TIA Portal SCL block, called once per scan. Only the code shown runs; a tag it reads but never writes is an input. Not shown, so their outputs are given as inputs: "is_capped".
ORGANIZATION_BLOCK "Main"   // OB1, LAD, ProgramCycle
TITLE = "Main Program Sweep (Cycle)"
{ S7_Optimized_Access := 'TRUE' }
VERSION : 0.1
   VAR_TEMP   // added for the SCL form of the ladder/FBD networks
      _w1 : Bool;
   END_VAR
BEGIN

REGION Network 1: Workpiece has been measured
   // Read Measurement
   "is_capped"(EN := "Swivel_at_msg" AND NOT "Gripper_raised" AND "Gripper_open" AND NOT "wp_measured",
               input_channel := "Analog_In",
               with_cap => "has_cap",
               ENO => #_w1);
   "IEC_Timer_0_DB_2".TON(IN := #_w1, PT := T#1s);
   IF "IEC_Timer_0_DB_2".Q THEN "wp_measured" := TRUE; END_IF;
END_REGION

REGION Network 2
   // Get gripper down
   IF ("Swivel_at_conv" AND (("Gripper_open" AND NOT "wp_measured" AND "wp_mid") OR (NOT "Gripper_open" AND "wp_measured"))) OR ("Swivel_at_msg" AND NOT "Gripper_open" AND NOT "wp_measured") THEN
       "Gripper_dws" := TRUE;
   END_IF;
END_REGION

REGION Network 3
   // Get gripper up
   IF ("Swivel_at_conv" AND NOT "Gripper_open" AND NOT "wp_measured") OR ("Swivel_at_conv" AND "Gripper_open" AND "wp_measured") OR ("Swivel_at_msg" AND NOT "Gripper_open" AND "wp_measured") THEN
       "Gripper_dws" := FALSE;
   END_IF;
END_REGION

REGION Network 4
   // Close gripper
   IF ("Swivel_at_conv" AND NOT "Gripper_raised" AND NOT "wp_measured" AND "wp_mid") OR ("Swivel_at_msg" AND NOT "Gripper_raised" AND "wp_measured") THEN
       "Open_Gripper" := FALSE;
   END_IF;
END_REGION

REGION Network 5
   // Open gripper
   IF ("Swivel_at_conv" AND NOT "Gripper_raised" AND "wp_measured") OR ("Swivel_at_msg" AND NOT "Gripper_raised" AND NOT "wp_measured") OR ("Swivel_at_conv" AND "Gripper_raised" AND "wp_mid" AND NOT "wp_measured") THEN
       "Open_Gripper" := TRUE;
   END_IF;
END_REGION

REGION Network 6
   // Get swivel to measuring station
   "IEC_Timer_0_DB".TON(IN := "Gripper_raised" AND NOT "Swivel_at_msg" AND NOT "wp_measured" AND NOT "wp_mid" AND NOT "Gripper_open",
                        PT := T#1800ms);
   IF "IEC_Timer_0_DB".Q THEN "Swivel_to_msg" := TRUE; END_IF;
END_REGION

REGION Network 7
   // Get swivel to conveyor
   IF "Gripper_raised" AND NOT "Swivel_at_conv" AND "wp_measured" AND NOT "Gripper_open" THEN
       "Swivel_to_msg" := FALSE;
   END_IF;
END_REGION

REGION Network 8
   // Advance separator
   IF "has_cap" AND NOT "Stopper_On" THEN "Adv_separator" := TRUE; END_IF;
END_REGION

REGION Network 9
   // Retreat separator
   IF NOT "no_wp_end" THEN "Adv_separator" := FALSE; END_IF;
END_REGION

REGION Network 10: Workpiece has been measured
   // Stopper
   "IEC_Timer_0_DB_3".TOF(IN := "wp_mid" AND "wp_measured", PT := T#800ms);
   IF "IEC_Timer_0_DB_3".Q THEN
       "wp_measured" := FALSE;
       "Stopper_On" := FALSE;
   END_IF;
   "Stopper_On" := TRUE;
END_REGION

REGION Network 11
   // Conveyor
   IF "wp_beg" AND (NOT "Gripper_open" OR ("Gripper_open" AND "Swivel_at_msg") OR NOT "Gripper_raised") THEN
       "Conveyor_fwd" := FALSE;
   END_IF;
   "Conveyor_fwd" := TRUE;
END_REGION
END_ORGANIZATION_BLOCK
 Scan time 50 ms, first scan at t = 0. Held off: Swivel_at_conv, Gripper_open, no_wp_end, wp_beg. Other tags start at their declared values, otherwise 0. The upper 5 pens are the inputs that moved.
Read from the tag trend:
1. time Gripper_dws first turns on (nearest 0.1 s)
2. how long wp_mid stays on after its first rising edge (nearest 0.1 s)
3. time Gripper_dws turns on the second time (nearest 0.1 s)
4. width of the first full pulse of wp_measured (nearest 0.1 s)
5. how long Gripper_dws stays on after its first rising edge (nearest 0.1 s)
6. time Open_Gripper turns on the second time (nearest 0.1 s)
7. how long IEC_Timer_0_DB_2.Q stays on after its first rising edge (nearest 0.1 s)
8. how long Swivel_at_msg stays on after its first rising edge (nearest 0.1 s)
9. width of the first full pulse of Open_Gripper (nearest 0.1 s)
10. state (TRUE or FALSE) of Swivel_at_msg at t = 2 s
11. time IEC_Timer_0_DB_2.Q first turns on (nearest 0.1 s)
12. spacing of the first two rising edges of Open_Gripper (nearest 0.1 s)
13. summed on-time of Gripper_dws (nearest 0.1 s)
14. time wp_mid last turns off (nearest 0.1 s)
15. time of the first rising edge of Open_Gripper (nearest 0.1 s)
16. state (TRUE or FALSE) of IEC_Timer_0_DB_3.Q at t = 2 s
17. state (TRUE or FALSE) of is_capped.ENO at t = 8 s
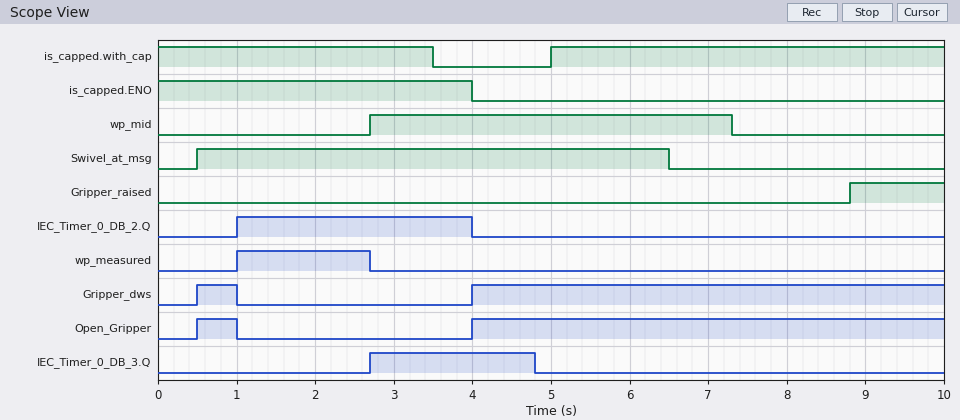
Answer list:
0.5 s
4.6 s
4.0 s
1.7 s
0.5 s
4.0 s
3.0 s
6.0 s
0.5 s
TRUE
1.0 s
3.5 s
6.5 s
7.3 s
0.5 s
FALSE
FALSE
